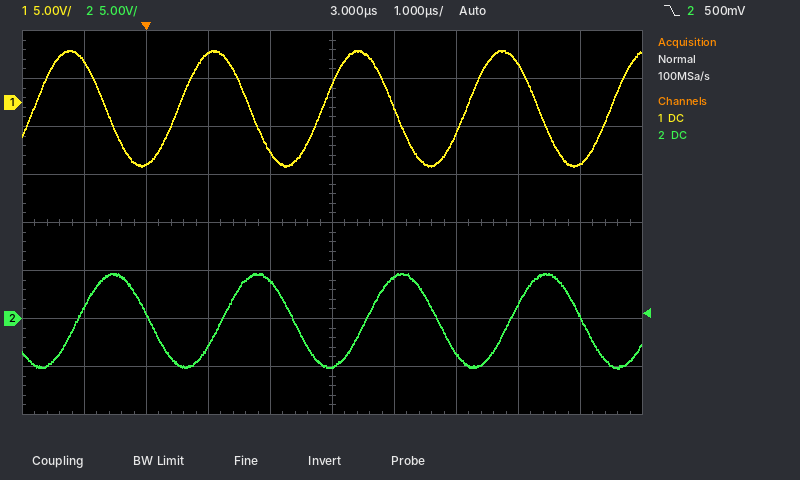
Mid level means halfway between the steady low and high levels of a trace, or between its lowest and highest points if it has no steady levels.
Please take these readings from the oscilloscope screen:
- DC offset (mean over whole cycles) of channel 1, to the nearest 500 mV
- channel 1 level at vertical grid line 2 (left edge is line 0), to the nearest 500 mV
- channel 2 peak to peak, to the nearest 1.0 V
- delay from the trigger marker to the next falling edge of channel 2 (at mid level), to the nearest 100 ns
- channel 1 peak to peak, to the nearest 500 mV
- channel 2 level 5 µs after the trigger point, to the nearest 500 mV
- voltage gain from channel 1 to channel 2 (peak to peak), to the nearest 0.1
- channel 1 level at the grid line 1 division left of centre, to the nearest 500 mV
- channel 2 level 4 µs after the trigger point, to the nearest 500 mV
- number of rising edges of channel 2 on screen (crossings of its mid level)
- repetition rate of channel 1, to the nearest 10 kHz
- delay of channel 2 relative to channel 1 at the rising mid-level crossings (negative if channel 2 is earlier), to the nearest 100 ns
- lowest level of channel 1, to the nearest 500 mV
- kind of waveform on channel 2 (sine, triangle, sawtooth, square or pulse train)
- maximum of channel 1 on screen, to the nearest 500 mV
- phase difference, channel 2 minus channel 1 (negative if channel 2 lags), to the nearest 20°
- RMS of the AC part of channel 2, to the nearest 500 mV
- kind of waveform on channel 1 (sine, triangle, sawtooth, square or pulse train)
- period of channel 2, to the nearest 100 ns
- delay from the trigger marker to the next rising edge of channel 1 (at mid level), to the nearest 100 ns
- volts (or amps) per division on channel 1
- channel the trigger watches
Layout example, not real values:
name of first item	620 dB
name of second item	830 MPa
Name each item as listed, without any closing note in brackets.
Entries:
DC offset (mean over whole cycles) of channel 1, to the nearest 500 mV	-500 mV
channel 1 level at vertical grid line 2 (left edge is line 0), to the nearest 500 mV	-6.5 V
channel 2 peak to peak, to the nearest 1.0 V	10.0 V
delay from the trigger marker to the next falling edge of channel 2 (at mid level), to the nearest 100 ns	100 ns
channel 1 peak to peak, to the nearest 500 mV	12.0 V
channel 2 level 5 µs after the trigger point, to the nearest 500 mV	-3.5 V
voltage gain from channel 1 to channel 2 (peak to peak), to the nearest 0.1	0.8
channel 1 level at the grid line 1 division left of centre, to the nearest 500 mV	-5.0 V
channel 2 level 4 µs after the trigger point, to the nearest 500 mV	4.5 V
number of rising edges of channel 2 on screen	4
repetition rate of channel 1, to the nearest 10 kHz	430 kHz
delay of channel 2 relative to channel 1 at the rising mid-level crossings (negative if channel 2 is earlier), to the nearest 100 ns	+700 ns
lowest level of channel 1, to the nearest 500 mV	-6.5 V
kind of waveform on channel 2	sine
maximum of channel 1 on screen, to the nearest 500 mV	5.5 V
phase difference, channel 2 minus channel 1 (negative if channel 2 lags), to the nearest 20°	-100°
RMS of the AC part of channel 2, to the nearest 500 mV	3.5 V
kind of waveform on channel 1	sine
period of channel 2, to the nearest 100 ns	2.3 µs
delay from the trigger marker to the next rising edge of channel 1 (at mid level), to the nearest 100 ns	500 ns
volts (or amps) per division on channel 1	5 V
channel the trigger watches	channel 2
